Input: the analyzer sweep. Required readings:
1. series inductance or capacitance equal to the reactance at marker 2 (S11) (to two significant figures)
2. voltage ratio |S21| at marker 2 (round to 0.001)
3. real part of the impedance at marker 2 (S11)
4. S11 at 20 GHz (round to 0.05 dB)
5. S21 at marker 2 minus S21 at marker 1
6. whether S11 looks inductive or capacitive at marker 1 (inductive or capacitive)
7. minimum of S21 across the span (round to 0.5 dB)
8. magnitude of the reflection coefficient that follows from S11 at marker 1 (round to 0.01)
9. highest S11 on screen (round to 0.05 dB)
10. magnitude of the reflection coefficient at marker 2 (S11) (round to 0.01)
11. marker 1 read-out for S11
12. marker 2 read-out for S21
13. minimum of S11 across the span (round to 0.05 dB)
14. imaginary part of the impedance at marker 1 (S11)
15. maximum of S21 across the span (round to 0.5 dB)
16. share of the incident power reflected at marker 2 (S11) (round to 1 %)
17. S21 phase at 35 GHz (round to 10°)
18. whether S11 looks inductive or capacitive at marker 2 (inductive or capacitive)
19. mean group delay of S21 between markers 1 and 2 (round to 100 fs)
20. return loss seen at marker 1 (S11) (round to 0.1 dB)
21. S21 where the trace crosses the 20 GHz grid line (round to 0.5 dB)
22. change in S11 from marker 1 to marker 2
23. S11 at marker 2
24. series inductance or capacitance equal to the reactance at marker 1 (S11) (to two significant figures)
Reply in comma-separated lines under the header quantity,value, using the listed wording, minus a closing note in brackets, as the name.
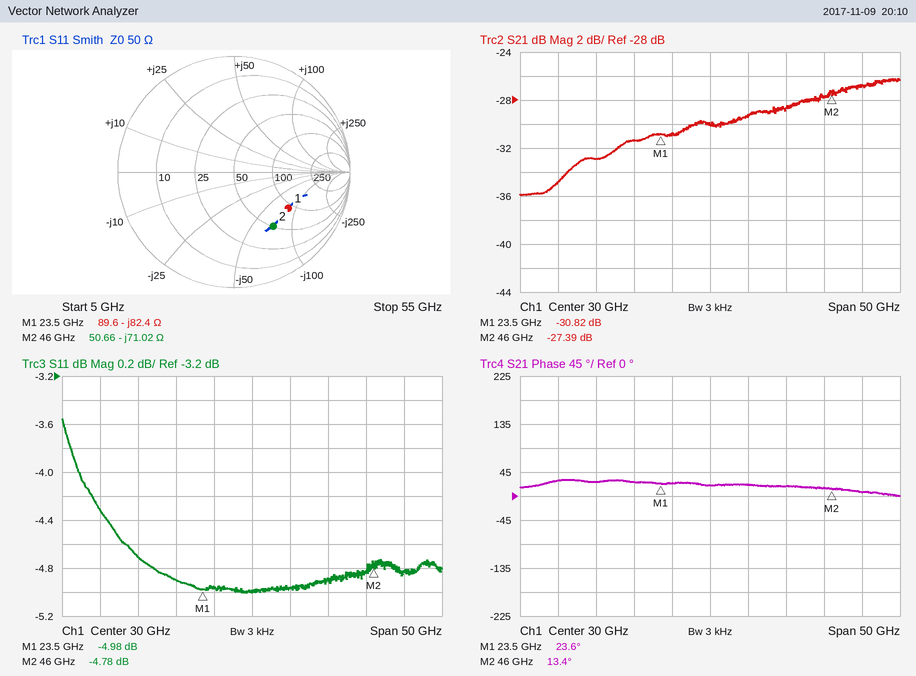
quantity,value
series inductance or capacitance equal to the reactance at marker 2 (S11),49 fF
voltage ratio |S21| at marker 2,0.043
real part of the impedance at marker 2,50.66 Ω
S11 at 20 GHz,-4.90 dB
S21 at marker 2 minus S21 at marker 1,3.43 dB
whether S11 looks inductive or capacitive at marker 1,capacitive
minimum of S21 across the span,-36.0 dB
magnitude of the reflection coefficient that follows from S11 at marker 1,0.56
highest S11 on screen,-3.55 dB
magnitude of the reflection coefficient at marker 2 (S11),0.58
marker 1 read-out for S11,-4.98 dB
marker 2 read-out for S21,-27.39 dB
minimum of S11 across the span,-5.00 dB
imaginary part of the impedance at marker 1,-82.4 Ω
maximum of S21 across the span,-26.0 dB
share of the incident power reflected at marker 2 (S11),33 %
S21 phase at 35 GHz,20°
whether S11 looks inductive or capacitive at marker 2,capacitive
mean group delay of S21 between markers 1 and 2,1.3 ps
return loss seen at marker 1 (S11),5.0 dB
S21 where the trace crosses the 20 GHz grid line,-31.5 dB
change in S11 from marker 1 to marker 2,0.20 dB
S11 at marker 2,-4.78 dB
series inductance or capacitance equal to the reactance at marker 1 (S11),82 fF
